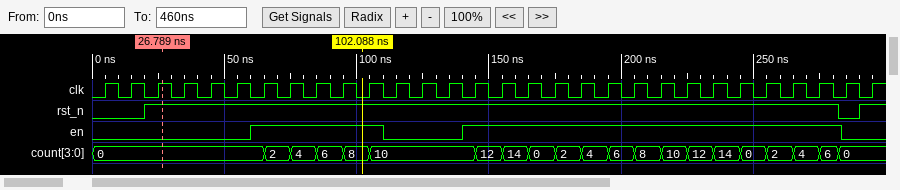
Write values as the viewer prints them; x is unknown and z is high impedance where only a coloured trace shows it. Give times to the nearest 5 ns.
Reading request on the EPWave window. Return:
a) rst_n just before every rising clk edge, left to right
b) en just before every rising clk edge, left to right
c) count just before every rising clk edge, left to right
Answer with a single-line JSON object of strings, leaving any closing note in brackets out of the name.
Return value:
{"rst_n just before every rising clk edge, left to right": "0 0 1 1 1 1 1 1 1 1 1 1 1 1 1 1 1 1 1 1 1 1 1 1 1 1 1 1 0 1", "en just before every rising clk edge, left to right": "0 0 0 0 0 0 1 1 1 1 1 0 0 0 1 1 1 1 1 1 1 1 1 1 1 1 1 1 0 0", "count just before every rising clk edge, left to right": "0, 0, 0, 0, 0, 0, 0, 2, 4, 6, 8, 10, 10, 10, 10, 12, 14, 0, 2, 4, 6, 8, 10, 12, 14, 0, 2, 4, 0, 0"}
